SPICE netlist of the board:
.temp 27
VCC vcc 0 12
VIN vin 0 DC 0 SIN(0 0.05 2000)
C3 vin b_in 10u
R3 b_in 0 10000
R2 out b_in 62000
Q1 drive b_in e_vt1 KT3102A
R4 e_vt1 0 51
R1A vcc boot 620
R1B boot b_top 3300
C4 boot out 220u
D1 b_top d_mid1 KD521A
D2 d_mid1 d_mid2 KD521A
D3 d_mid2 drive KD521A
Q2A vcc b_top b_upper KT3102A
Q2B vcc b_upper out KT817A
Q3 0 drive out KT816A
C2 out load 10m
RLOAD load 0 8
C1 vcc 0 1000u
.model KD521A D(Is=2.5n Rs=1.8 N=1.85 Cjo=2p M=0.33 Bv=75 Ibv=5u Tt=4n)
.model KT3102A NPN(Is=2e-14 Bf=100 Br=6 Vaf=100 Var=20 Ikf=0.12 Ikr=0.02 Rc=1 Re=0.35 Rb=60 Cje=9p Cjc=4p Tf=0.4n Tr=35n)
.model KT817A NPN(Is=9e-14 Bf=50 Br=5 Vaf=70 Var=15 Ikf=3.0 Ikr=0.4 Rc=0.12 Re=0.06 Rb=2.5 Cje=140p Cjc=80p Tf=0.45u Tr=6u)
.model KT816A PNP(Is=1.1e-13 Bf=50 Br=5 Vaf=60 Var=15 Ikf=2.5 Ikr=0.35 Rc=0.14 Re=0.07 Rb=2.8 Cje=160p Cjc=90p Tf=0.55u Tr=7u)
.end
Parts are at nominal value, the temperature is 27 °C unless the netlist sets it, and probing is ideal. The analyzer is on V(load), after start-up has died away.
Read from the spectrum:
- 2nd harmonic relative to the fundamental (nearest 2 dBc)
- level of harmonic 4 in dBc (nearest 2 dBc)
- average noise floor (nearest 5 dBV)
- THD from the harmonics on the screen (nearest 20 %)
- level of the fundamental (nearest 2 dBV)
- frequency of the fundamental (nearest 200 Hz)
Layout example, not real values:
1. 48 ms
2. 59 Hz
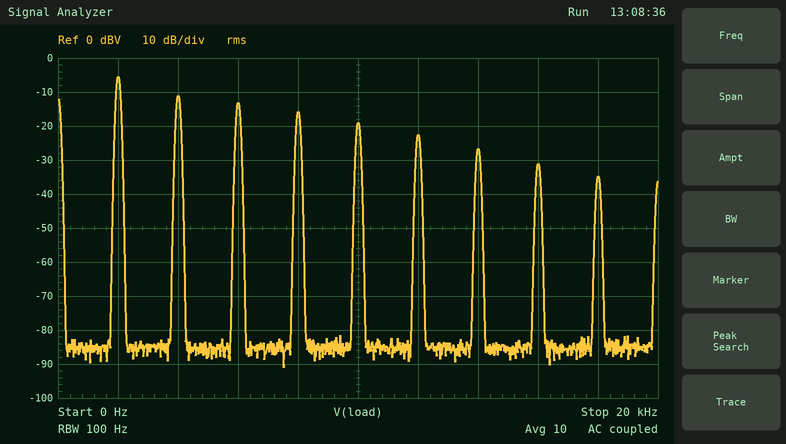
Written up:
1. -6 dBc
2. -10 dBc
3. -85 dBV
4. 80 %
5. -6 dBV
6. 2.0 kHz
